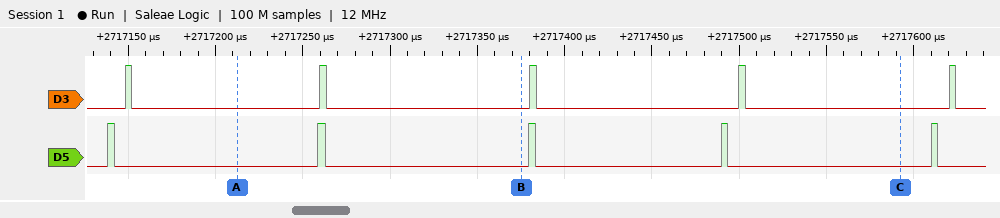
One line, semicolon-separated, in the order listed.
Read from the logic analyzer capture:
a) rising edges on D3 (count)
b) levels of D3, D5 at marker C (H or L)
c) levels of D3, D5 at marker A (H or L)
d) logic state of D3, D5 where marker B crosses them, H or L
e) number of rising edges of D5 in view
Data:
5; D3=L, D5=L; D3=L, D5=L; D3=L, D5=L; 5
